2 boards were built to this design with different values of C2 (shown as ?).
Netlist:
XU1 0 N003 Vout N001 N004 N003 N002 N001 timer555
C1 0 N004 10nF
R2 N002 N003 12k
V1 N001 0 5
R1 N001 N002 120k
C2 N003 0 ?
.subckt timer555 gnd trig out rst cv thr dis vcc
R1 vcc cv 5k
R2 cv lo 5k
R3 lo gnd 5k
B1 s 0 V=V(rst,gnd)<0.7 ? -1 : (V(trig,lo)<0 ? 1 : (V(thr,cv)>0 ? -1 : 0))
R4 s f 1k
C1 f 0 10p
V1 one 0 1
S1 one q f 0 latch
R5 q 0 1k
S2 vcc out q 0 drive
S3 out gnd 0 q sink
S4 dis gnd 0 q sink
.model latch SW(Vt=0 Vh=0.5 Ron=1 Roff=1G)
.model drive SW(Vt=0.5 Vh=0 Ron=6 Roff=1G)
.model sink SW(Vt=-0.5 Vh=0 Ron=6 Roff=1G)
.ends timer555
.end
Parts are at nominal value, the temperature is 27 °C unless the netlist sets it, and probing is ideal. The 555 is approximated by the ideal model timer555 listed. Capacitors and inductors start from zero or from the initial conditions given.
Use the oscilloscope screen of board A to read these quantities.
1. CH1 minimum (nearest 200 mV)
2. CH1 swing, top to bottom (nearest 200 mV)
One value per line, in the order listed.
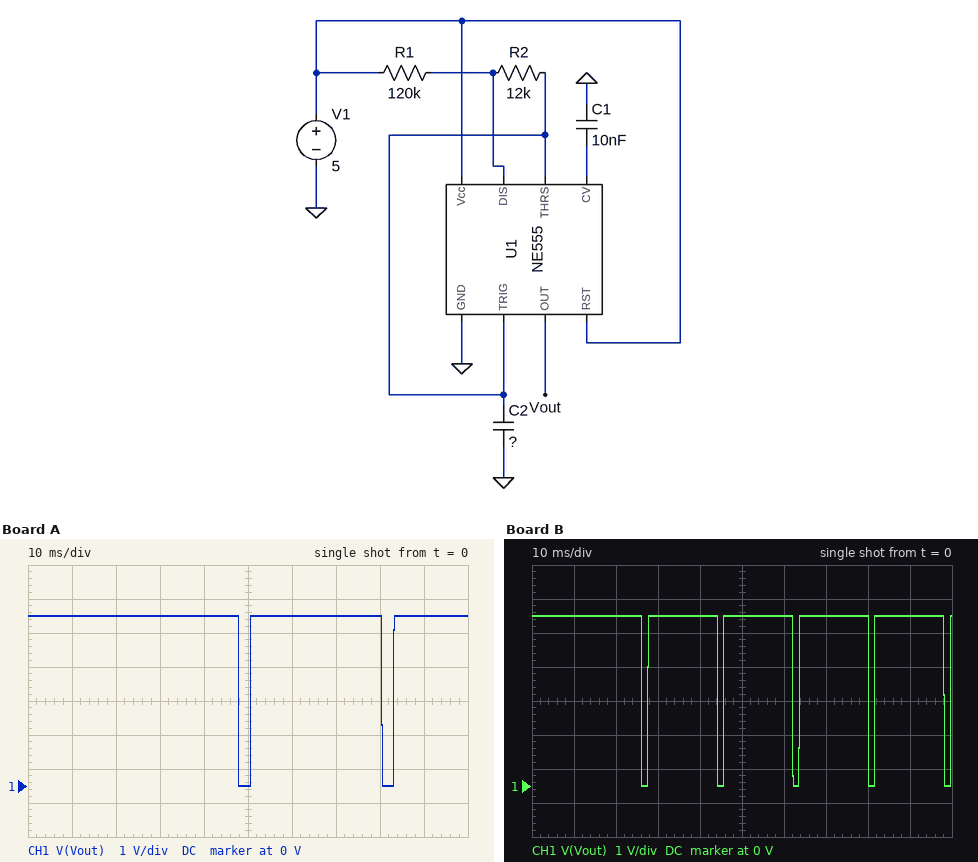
0 V
5.0 V
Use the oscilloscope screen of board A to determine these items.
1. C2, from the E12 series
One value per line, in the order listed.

330 nF
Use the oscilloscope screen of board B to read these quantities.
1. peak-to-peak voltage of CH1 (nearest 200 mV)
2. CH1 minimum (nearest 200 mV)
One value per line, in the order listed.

5.0 V
0 V
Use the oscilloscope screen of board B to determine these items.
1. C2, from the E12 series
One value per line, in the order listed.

180 nF
